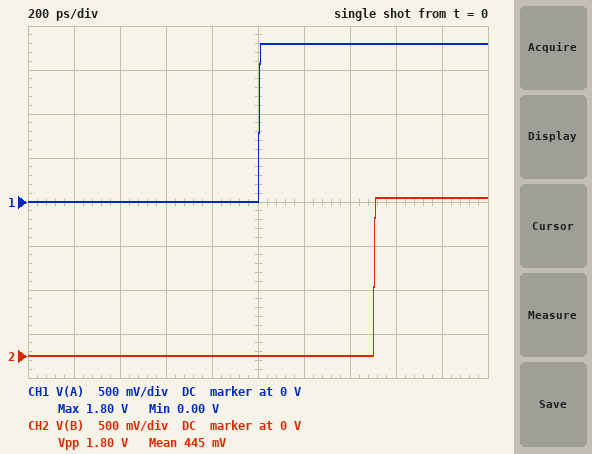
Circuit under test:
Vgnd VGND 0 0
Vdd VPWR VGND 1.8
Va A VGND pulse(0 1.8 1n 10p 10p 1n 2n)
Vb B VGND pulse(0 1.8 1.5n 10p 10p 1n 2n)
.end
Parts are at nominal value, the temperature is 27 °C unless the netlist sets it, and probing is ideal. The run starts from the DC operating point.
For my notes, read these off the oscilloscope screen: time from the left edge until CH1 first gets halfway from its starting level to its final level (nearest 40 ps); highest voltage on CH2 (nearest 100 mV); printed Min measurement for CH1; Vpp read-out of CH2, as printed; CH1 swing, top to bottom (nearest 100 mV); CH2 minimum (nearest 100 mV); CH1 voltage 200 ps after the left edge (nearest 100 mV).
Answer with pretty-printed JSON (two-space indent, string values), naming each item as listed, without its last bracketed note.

{
  "time from the left edge until CH1 first gets halfway from its starting level to its final level": "1.00 ns",
  "highest voltage on CH2": "1.8 V",
  "printed Min measurement for CH1": "0.00 V",
  "Vpp read-out of CH2, as printed": "1.80 V",
  "CH1 swing, top to bottom": "1.8 V",
  "CH2 minimum": "0 V",
  "CH1 voltage 200 ps after the left edge": "0 V"
}
